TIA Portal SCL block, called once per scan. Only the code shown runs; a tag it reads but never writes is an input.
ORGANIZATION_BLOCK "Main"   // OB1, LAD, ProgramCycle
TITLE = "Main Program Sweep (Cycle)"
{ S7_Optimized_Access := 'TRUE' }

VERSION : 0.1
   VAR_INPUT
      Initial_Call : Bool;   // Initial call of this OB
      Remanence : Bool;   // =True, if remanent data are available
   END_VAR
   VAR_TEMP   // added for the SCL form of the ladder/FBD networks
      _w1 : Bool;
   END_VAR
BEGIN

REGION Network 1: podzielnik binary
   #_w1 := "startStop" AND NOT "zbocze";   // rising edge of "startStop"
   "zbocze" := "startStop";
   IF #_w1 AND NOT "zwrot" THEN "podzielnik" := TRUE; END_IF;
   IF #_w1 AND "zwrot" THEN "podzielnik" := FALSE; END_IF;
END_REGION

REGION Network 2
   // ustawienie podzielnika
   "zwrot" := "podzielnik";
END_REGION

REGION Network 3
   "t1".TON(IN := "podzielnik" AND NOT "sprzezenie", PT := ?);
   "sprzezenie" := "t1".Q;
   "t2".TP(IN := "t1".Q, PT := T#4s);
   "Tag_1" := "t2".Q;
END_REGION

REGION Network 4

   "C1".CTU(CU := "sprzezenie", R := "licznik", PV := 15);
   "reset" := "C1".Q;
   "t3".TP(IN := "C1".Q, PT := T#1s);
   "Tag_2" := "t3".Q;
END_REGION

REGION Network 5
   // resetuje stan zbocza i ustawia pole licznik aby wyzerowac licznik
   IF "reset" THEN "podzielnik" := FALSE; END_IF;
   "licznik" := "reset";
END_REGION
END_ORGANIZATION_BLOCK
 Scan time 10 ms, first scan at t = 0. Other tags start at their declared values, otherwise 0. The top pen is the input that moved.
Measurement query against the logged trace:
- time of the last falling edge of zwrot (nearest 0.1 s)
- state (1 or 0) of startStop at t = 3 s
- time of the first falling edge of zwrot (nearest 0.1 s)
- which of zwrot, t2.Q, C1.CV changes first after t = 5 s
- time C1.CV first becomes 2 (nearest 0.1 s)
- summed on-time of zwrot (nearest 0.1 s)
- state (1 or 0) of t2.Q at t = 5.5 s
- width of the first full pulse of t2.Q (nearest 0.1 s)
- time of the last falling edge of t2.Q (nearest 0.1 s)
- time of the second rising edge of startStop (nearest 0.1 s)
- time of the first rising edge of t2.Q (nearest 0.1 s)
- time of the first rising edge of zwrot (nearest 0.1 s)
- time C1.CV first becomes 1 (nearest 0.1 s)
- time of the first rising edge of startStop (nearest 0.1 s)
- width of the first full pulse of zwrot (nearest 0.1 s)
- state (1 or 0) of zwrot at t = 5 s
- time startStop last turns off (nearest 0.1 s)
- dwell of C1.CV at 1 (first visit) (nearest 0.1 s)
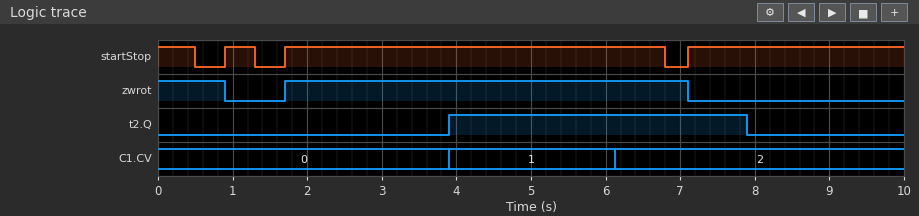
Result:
7.1 s
1
0.9 s
C1.CV
6.1 s
6.3 s
1
4.0 s
7.9 s
1.7 s
3.9 s
1.7 s
3.9 s
0.9 s
5.4 s
1
6.8 s
2.2 s
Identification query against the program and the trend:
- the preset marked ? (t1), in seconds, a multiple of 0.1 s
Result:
2.2 s
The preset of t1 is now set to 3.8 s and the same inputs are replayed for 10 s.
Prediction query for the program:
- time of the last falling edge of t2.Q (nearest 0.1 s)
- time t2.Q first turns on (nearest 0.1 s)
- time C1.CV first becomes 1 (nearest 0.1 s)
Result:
9.5 s
5.5 s
5.5 s
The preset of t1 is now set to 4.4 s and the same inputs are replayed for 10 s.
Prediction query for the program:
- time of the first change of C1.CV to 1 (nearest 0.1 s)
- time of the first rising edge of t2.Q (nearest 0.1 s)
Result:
6.1 s
6.1 s
